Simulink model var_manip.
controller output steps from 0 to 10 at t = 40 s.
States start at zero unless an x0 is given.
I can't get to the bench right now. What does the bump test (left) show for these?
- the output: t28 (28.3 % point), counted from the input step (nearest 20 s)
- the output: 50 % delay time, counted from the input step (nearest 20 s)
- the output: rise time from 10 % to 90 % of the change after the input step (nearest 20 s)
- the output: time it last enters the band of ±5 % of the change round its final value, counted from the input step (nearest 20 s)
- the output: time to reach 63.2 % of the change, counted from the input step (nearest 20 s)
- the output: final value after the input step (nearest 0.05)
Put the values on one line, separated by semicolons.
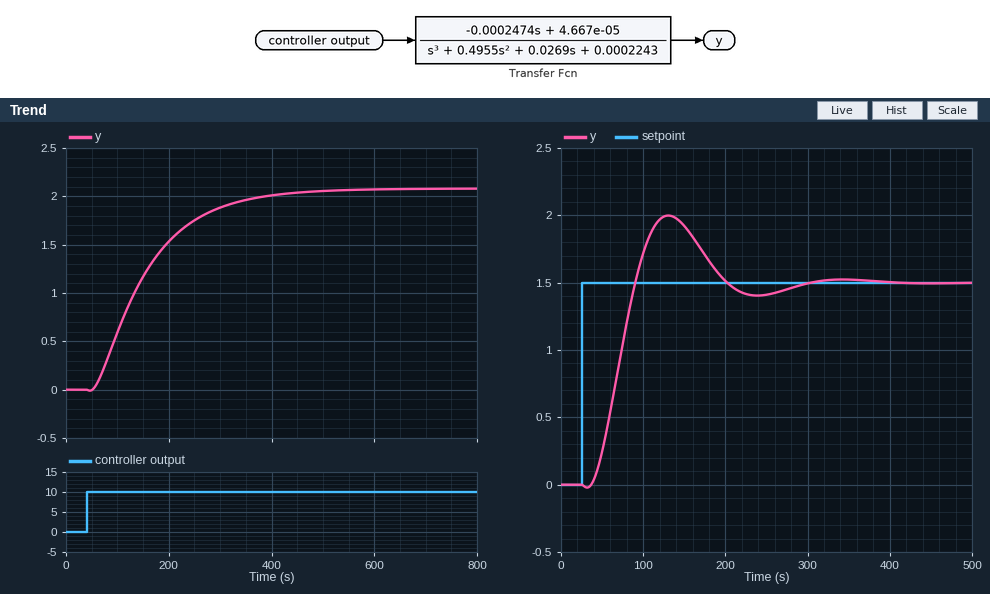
60 s; 100 s; 220 s; 320 s; 120 s; 2.10
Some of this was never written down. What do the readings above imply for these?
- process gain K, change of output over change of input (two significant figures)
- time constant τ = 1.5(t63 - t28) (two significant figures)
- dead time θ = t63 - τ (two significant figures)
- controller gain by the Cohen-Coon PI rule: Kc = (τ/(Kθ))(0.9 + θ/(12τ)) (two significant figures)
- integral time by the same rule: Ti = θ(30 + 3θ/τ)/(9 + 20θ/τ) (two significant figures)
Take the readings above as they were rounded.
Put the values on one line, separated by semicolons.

0.21; 90 s; 30 s; 13; 59 s
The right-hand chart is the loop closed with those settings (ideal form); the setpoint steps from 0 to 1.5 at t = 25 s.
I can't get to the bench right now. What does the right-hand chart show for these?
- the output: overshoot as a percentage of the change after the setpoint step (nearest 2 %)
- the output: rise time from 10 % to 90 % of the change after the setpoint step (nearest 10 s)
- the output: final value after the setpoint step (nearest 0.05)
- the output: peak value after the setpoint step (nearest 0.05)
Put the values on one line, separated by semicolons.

34 %; 40 s; 1.50; 2.00
